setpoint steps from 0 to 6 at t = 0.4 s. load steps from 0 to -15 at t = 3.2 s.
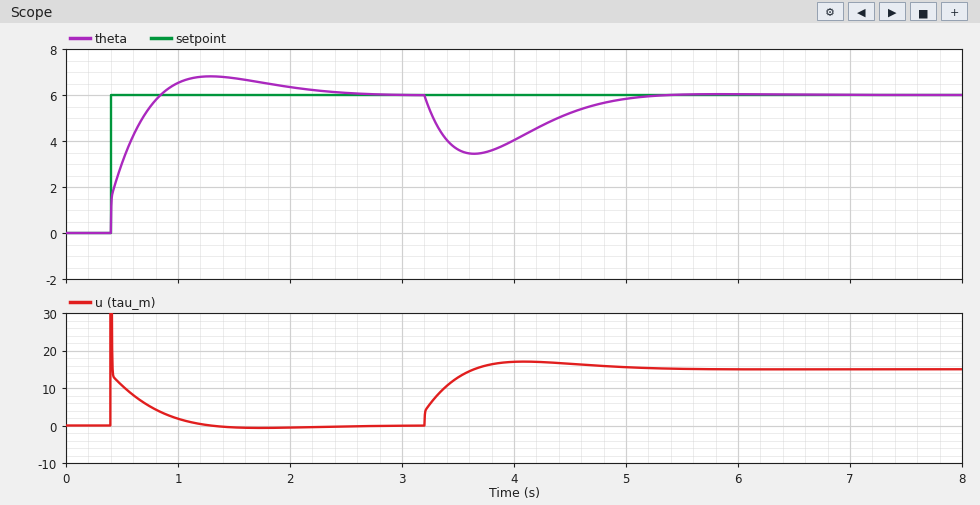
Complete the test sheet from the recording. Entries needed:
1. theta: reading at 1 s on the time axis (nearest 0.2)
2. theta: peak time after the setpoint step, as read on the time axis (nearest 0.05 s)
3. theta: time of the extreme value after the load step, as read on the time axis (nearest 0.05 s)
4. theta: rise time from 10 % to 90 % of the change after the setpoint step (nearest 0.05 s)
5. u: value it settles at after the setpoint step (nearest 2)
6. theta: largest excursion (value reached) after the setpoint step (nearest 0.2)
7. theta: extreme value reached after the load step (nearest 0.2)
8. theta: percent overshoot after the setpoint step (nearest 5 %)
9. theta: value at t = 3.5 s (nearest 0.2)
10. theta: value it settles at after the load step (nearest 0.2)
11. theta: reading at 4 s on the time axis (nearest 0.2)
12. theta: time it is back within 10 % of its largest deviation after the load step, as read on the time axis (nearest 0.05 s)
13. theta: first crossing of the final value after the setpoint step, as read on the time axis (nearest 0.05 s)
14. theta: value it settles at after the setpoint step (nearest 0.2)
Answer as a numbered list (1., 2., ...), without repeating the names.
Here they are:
1. 6.6
2. 1.30 s
3. 3.65 s
4. 0.35 s
5. 0
6. 6.8
7. 3.4
8. 15 %
9. 3.6
10. 6.0
11. 4.0
12. 4.90 s
13. 0.85 s
14. 6.0
